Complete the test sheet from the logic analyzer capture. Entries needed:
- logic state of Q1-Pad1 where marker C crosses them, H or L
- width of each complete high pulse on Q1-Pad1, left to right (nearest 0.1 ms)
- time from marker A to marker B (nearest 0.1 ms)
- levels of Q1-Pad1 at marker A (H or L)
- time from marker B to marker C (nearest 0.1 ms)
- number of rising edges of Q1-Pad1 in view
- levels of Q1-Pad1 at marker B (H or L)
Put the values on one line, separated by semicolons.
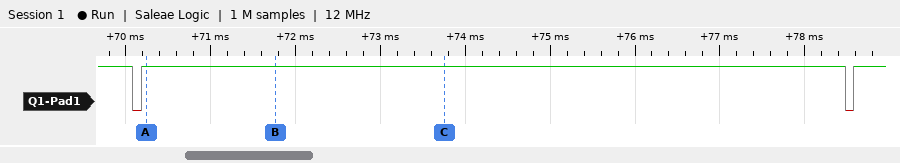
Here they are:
Q1-Pad1=H; 8.3 ms; 1.5 ms; Q1-Pad1=H; 2 ms; 2; Q1-Pad1=H
